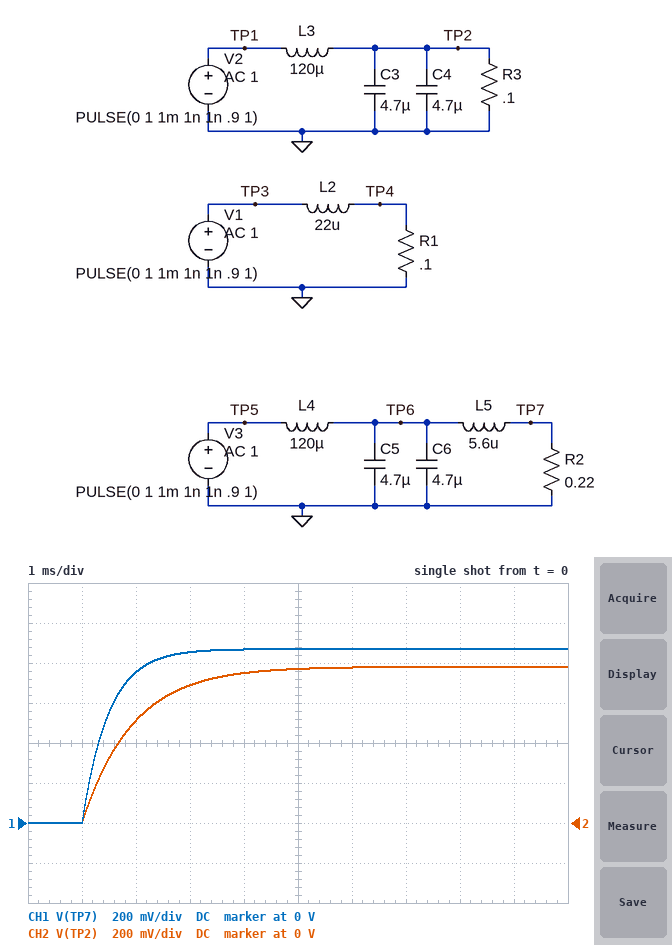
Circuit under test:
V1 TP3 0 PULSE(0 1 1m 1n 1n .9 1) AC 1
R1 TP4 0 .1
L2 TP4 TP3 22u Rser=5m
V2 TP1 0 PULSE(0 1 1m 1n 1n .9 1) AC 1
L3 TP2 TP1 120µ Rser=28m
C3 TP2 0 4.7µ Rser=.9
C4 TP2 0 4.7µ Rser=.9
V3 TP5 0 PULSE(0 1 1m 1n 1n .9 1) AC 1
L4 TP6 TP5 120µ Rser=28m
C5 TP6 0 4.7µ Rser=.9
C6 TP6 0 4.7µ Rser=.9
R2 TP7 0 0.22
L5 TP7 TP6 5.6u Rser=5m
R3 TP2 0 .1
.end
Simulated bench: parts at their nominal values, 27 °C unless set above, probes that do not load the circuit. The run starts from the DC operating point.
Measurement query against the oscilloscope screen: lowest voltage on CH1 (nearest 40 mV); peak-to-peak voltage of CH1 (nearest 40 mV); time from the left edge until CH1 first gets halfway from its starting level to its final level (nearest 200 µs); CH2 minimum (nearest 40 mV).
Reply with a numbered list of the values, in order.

1. 0 V
2. 880 mV
3. 1.4 ms
4. 0 V
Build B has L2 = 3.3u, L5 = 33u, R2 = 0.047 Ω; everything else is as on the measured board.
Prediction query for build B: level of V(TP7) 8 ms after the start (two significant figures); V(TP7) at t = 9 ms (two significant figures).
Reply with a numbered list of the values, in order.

1. 570 mV
2. 580 mV
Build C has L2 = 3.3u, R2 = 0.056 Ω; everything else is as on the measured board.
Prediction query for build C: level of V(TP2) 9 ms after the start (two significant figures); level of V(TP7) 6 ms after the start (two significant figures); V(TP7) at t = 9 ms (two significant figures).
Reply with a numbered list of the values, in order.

1. 780 mV
2. 610 mV
3. 630 mV
